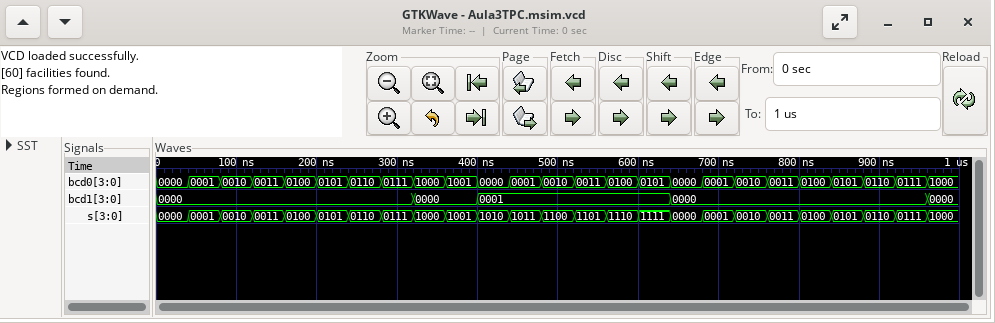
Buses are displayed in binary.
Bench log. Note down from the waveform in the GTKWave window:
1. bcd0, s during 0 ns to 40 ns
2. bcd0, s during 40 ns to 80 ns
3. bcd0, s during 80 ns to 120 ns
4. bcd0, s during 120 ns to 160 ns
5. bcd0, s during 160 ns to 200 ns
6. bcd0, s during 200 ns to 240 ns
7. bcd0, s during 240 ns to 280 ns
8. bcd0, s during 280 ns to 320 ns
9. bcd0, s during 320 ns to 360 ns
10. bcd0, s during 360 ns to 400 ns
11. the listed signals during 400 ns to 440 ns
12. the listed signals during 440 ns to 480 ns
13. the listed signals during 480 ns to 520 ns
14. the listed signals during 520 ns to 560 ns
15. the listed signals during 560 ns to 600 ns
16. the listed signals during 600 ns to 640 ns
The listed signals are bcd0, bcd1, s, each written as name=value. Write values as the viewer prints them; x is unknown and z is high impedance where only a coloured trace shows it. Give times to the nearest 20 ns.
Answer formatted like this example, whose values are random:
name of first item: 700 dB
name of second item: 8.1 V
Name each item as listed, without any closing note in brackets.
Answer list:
bcd0, s during 0 ns to 40 ns: bcd0=0000, s=0000
bcd0, s during 40 ns to 80 ns: bcd0=0001, s=0001
bcd0, s during 80 ns to 120 ns: bcd0=0010, s=0010
bcd0, s during 120 ns to 160 ns: bcd0=0011, s=0011
bcd0, s during 160 ns to 200 ns: bcd0=0100, s=0100
bcd0, s during 200 ns to 240 ns: bcd0=0101, s=0101
bcd0, s during 240 ns to 280 ns: bcd0=0110, s=0110
bcd0, s during 280 ns to 320 ns: bcd0=0111, s=0111
bcd0, s during 320 ns to 360 ns: bcd0=1000, s=1000
bcd0, s during 360 ns to 400 ns: bcd0=1001, s=1001
the listed signals during 400 ns to 440 ns: bcd0=0000, bcd1=0001, s=1010
the listed signals during 440 ns to 480 ns: bcd0=0001, bcd1=0001, s=1011
the listed signals during 480 ns to 520 ns: bcd0=0010, bcd1=0001, s=1100
the listed signals during 520 ns to 560 ns: bcd0=0011, bcd1=0001, s=1101
the listed signals during 560 ns to 600 ns: bcd0=0100, bcd1=0001, s=1110
the listed signals during 600 ns to 640 ns: bcd0=0101, bcd1=0001, s=1111
